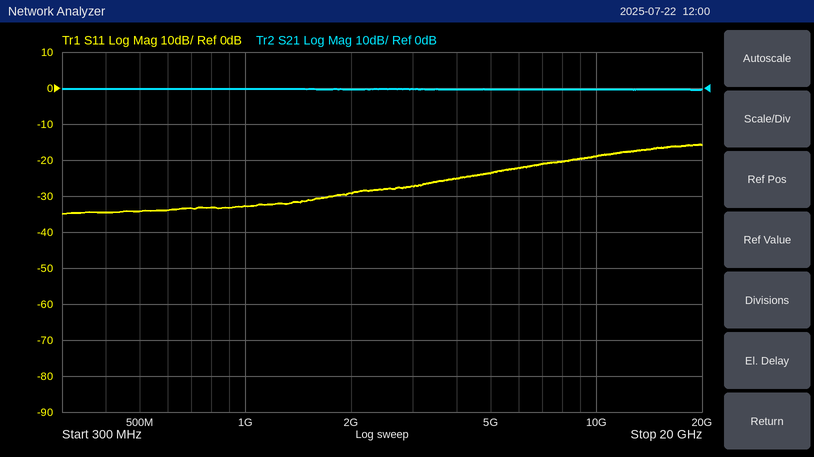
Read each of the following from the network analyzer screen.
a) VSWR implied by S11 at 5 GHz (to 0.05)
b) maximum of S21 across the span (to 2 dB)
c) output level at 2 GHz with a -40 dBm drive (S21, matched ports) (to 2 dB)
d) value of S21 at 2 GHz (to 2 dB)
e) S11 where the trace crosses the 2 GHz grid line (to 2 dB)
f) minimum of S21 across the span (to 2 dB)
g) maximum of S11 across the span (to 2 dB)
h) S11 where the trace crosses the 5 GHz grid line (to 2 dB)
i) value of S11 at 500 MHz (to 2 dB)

1.15
0 dB
-40 dBm
0 dB
-30 dB
0 dB
-16 dB
-24 dB
-34 dB
